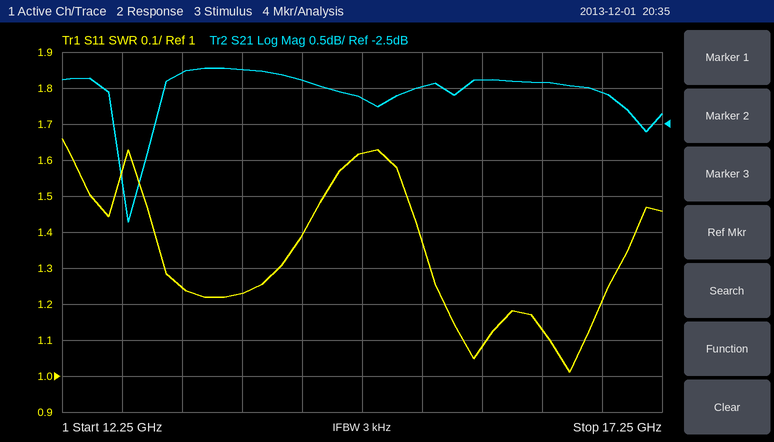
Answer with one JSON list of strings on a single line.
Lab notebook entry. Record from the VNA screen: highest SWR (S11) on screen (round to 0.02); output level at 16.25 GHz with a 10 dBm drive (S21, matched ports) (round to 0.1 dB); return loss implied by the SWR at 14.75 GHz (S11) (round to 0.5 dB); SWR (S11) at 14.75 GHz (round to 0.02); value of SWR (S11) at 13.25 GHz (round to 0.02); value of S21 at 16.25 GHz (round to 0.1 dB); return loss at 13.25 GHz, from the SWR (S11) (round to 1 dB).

["1.66", "8.1 dBm", "12.5 dB", "1.62", "1.24", "-1.9 dB", "19 dB"]
